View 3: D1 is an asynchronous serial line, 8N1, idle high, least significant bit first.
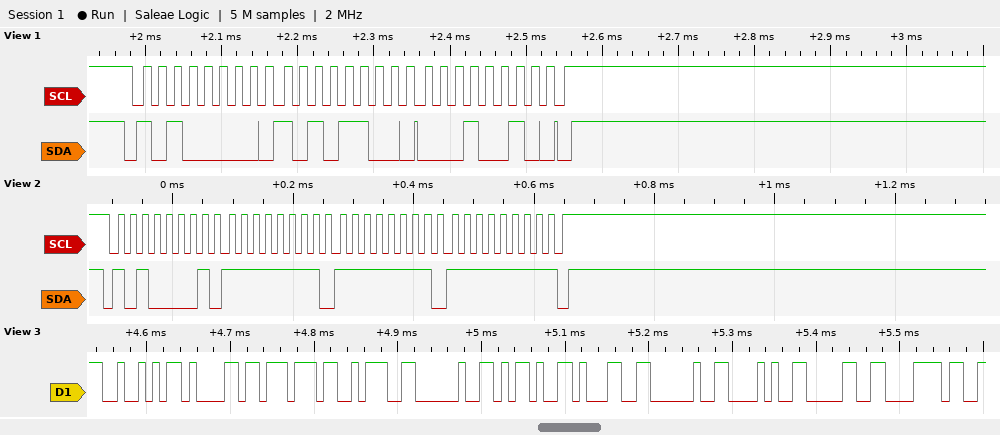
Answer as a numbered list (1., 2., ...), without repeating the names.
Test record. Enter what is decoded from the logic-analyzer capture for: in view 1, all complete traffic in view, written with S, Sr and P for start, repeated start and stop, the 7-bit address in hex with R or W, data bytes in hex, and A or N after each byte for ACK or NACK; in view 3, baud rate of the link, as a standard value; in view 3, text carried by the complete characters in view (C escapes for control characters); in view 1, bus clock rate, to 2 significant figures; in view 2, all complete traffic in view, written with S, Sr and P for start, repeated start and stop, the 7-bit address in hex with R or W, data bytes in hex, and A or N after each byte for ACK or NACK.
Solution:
1. S 50W A AC A 12 A P
2. 115200 baud
3. "Raw: -1 (0x"
4. 50 kHz
5. S 50R A FF A FF A FF N P
